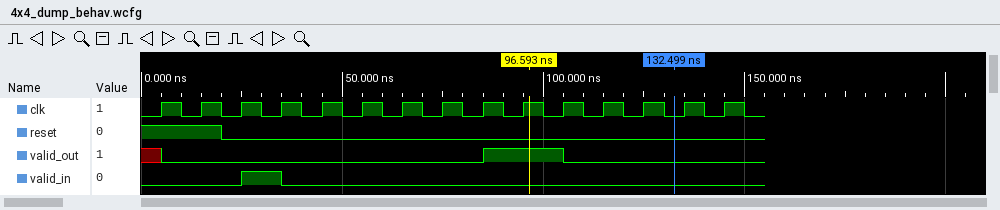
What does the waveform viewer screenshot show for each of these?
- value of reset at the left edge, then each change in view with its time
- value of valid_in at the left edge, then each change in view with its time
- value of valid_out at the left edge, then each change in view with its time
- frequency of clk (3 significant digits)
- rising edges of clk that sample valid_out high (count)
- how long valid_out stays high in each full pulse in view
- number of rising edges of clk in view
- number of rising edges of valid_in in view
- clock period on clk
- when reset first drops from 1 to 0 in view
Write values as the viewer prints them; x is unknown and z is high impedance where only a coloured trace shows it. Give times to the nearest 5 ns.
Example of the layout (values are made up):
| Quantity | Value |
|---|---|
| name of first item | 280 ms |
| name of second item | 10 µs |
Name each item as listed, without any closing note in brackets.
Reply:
| Quantity | Value |
|---|---|
| value of reset at the left edge, then each change in view with its time | 1, 0 at 20 ns |
| value of valid_in at the left edge, then each change in view with its time | 0, 1 at 25 ns, 0 at 35 ns |
| value of valid_out at the left edge, then each change in view with its time | x, 0 at 5 ns, 1 at 85 ns, 0 at 105 ns |
| frequency of clk | 100 MHz |
| rising edges of clk that sample valid_out high | 2 |
| how long valid_out stays high in each full pulse in view | 20 ns |
| number of rising edges of clk in view | 15 |
| number of rising edges of valid_in in view | 1 |
| clock period on clk | 10 ns |
| when reset first drops from 1 to 0 in view | 20 ns |
